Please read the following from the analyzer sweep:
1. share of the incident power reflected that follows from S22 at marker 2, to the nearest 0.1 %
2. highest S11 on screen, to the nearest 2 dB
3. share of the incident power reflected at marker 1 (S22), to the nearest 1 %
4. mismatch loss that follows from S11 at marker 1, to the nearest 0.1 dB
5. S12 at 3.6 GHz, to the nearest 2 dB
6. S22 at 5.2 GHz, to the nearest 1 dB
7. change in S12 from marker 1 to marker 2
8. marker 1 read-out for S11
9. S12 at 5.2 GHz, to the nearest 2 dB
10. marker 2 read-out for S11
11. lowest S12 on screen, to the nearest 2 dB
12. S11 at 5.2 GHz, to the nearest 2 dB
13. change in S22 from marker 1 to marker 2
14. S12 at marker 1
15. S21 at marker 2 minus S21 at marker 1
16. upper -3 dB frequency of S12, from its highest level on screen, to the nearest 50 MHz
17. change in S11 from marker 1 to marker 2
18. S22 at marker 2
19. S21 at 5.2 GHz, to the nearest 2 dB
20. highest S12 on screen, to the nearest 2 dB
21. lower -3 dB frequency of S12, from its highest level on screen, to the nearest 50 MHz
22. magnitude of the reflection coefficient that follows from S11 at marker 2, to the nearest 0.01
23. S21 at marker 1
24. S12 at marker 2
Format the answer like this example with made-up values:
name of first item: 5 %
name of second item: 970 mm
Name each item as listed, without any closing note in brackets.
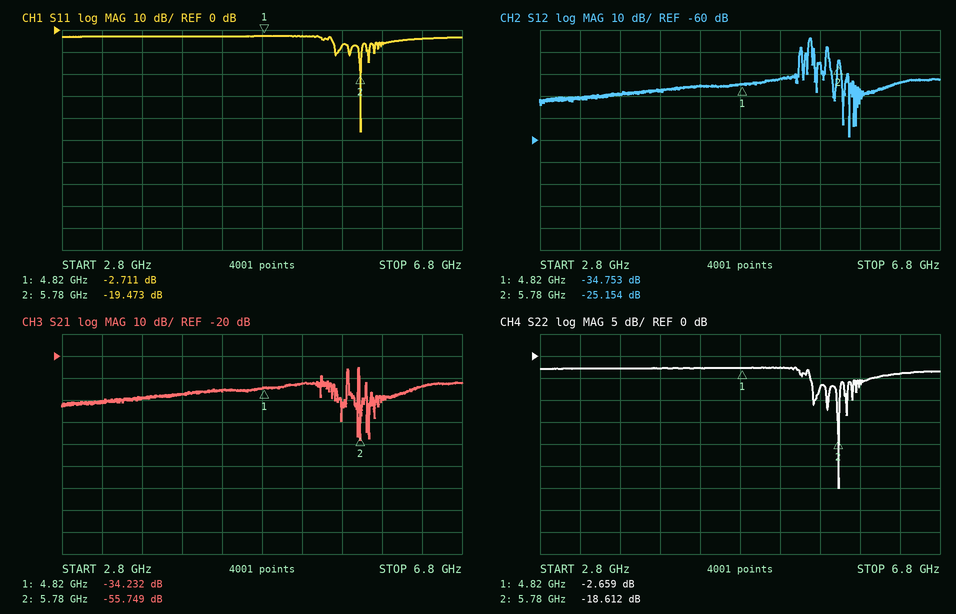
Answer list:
share of the incident power reflected that follows from S22 at marker 2, to the nearest 0.1 %: 1.4 %
highest S11 on screen, to the nearest 2 dB: -2 dB
share of the incident power reflected at marker 1 (S22), to the nearest 1 %: 54 %
mismatch loss that follows from S11 at marker 1, to the nearest 0.1 dB: 3.3 dB
S12 at 3.6 GHz, to the nearest 2 dB: -40 dB
S22 at 5.2 GHz, to the nearest 1 dB: -3 dB
change in S12 from marker 1 to marker 2: 9.599 dB
marker 1 read-out for S11: -2.711 dB
S12 at 5.2 GHz, to the nearest 2 dB: -32 dB
marker 2 read-out for S11: -19.473 dB
lowest S12 on screen, to the nearest 2 dB: -58 dB
S11 at 5.2 GHz, to the nearest 2 dB: -2 dB
change in S22 from marker 1 to marker 2: -15.953 dB
S12 at marker 1: -34.753 dB
S21 at marker 2 minus S21 at marker 1: -21.517 dB
upper -3 dB frequency of S12, from its highest level on screen, to the nearest 50 MHz: 5.50 GHz
change in S11 from marker 1 to marker 2: -16.762 dB
S22 at marker 2: -18.612 dB
S21 at 5.2 GHz, to the nearest 2 dB: -32 dB
highest S12 on screen, to the nearest 2 dB: -14 dB
lower -3 dB frequency of S12, from its highest level on screen, to the nearest 50 MHz: 5.50 GHz
magnitude of the reflection coefficient that follows from S11 at marker 2, to the nearest 0.01: 0.11
S21 at marker 1: -34.232 dB
S12 at marker 2: -25.154 dB
